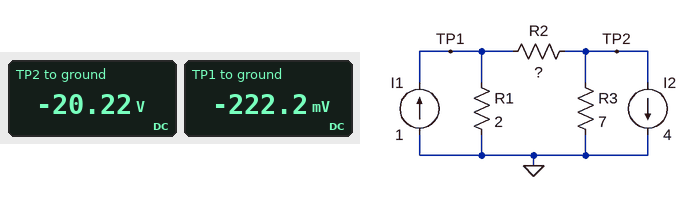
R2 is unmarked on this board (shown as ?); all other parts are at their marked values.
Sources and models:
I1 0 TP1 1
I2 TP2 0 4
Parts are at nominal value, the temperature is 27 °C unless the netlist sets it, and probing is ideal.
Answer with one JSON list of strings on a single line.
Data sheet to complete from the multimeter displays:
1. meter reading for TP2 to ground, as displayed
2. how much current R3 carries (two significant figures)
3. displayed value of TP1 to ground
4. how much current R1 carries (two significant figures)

["-20.22 V", "2.9 A", "-222.2 mV", "110 mA"]
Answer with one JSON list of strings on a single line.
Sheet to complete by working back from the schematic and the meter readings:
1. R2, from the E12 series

["18 Ω"]
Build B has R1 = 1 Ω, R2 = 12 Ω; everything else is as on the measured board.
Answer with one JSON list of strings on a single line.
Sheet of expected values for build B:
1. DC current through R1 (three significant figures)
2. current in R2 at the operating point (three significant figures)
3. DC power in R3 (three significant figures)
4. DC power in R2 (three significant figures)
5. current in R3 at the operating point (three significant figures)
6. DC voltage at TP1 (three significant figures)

["450 mA", "1.45 A", "45.5 W", "25.2 W", "2.55 A", "-450 mV"]
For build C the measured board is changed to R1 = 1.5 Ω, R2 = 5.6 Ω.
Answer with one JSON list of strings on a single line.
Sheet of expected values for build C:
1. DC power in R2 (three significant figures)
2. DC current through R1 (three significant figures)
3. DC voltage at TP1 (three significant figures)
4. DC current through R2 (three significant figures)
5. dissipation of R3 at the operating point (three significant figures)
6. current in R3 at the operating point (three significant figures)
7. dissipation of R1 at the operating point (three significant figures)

["24.5 W", "1.09 A", "-1.64 V", "2.09 A", "25.5 W", "1.91 A", "1.79 W"]
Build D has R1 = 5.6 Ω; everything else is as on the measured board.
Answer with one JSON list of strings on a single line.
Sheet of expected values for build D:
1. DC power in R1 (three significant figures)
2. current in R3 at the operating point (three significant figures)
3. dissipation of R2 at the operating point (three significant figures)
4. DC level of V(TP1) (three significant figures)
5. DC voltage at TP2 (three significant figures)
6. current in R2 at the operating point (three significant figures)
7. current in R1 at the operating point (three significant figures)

["53.8 mW", "2.90 A", "21.7 W", "-549 mV", "-20.3 V", "1.10 A", "98.0 mA"]
